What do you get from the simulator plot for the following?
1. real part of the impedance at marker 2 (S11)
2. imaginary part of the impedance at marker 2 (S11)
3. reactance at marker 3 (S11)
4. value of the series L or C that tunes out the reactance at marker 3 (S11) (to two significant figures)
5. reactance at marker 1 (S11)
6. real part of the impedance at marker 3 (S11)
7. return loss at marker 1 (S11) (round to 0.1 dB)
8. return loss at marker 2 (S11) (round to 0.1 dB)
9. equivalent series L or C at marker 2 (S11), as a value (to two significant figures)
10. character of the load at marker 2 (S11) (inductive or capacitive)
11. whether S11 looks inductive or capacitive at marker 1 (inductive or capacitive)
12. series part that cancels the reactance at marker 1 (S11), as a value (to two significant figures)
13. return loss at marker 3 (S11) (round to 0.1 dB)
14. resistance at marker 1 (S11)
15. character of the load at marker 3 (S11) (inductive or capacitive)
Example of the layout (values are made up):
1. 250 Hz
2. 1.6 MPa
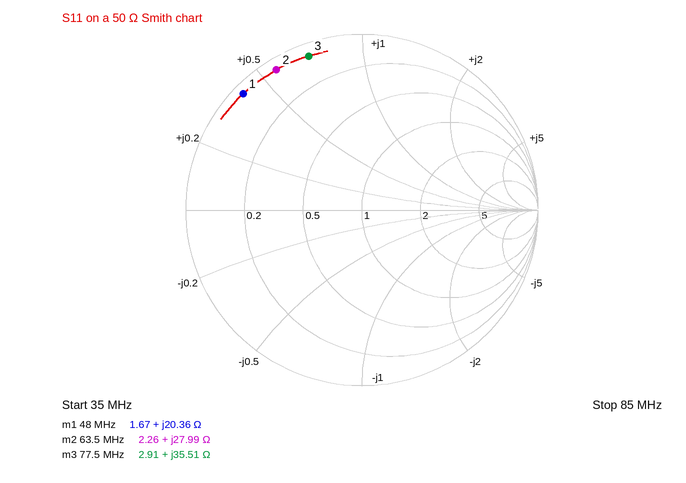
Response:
1. 2.26 Ω
2. +27.99 Ω
3. +35.51 Ω
4. 58 pF
5. +20.36 Ω
6. 2.91 Ω
7. 0.5 dB
8. 0.6 dB
9. 70 nH
10. inductive
11. inductive
12. 160 pF
13. 0.7 dB
14. 1.67 Ω
15. inductive
